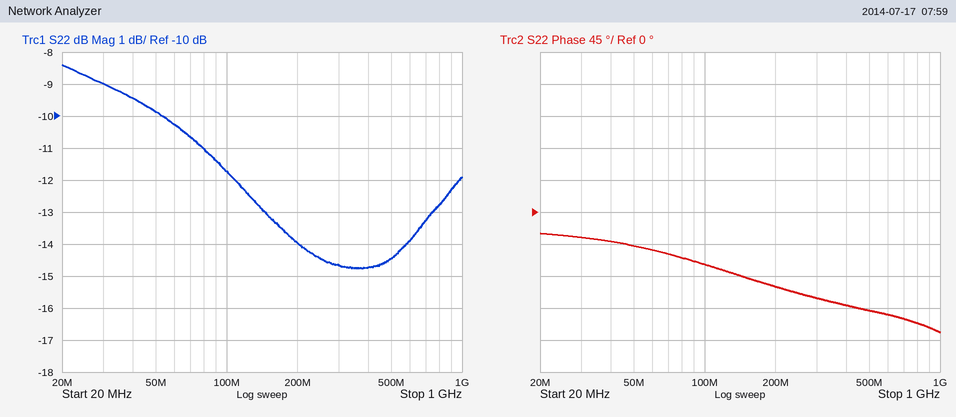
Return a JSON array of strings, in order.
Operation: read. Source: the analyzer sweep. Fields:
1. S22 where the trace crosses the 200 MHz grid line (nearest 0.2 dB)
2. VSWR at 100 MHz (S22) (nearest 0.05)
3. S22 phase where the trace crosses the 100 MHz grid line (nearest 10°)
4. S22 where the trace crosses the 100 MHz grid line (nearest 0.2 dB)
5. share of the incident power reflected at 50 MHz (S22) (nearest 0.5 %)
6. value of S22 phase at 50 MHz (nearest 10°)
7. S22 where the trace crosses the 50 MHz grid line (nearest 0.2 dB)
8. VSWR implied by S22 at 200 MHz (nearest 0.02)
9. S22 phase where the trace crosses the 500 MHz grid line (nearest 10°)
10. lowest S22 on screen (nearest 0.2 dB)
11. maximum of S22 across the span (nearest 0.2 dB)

["-14.0 dB", "1.70", "-70°", "-11.8 dB", "10.5 %", "-50°", "-9.8 dB", "1.50", "-140°", "-14.8 dB", "-8.4 dB"]
